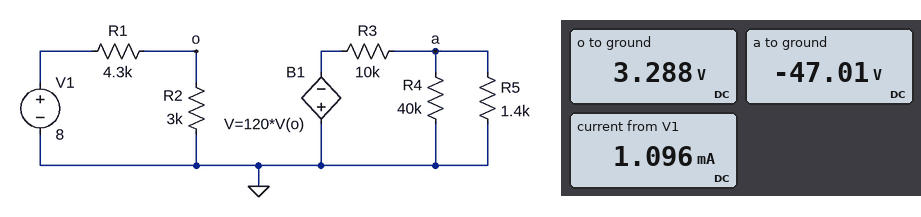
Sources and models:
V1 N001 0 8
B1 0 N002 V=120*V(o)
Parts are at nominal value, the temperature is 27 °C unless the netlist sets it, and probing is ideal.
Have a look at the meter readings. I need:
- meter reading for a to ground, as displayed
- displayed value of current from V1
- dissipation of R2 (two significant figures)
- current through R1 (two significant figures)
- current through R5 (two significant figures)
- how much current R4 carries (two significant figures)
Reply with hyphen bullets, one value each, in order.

- -47.01 V
- 1.096 mA
- 3.6 mW
- 1.1 mA
- 34 mA
- 1.2 mA
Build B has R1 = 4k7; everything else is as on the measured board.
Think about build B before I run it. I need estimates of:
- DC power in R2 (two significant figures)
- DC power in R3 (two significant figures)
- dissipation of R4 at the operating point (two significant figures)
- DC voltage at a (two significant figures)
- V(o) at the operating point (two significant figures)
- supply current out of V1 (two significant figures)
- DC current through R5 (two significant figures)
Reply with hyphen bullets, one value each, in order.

- 3.2 mW
- 11 W
- 50 mW
- -45 V
- 3.1 V
- 1.0 mA
- 32 mA
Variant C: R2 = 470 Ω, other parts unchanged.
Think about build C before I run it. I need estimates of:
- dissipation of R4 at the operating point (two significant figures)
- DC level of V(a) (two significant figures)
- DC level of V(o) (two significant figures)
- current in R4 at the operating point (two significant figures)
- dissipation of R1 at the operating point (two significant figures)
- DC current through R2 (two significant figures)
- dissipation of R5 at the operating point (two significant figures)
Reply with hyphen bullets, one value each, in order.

- 3.2 mW
- -11 V
- 790 mV
- 280 µA
- 12 mW
- 1.7 mA
- 91 mW
